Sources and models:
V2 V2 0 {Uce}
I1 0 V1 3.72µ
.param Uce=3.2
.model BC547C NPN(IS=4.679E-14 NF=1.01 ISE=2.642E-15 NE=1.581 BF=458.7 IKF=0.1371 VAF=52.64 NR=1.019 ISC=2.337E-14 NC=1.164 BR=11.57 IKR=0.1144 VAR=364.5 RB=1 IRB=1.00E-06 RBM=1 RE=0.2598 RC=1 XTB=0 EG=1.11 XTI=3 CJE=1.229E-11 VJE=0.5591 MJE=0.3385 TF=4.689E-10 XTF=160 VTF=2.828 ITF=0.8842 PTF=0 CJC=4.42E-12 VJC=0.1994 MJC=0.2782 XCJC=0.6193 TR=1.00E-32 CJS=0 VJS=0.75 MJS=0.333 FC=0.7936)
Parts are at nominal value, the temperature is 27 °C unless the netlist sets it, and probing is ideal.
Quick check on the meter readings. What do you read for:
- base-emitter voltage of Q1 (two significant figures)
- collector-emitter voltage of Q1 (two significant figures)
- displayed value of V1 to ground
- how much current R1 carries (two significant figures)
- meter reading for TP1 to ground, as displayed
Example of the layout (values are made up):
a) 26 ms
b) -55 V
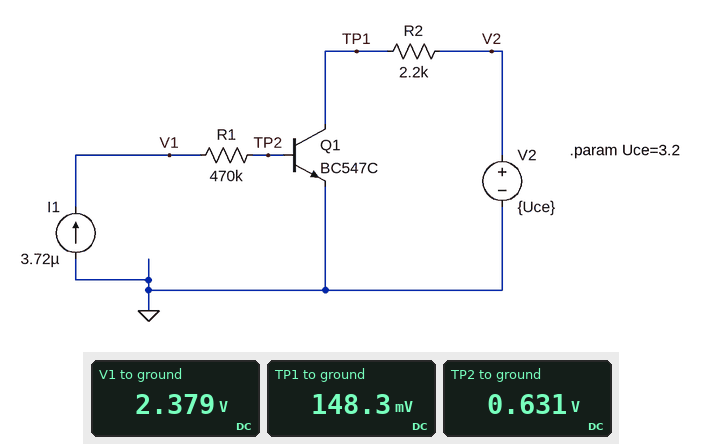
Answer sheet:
a) 630 mV
b) 150 mV
c) 2.379 V
d) 3.7 µA
e) 148.3 mV
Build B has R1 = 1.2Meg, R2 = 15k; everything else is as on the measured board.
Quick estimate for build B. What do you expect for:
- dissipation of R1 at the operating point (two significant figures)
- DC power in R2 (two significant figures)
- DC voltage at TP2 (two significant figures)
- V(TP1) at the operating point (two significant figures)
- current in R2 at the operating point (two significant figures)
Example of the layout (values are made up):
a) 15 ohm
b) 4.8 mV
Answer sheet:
a) 17 µW
b) 660 µW
c) 580 mV
d) 55 mV
e) 210 µA
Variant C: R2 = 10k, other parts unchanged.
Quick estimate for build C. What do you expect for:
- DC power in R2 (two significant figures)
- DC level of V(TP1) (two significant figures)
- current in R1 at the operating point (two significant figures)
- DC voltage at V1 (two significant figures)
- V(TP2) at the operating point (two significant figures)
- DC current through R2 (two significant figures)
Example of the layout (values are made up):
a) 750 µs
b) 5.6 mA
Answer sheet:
a) 980 µW
b) 66 mV
c) 3.7 µA
d) 2.3 V
e) 590 mV
f) 310 µA
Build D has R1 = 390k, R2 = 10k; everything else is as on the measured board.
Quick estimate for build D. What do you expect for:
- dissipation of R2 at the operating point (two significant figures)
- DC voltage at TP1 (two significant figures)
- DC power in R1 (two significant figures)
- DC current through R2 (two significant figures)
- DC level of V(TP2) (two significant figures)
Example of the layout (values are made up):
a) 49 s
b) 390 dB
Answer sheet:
a) 980 µW
b) 66 mV
c) 5.4 µW
d) 310 µA
e) 590 mV
